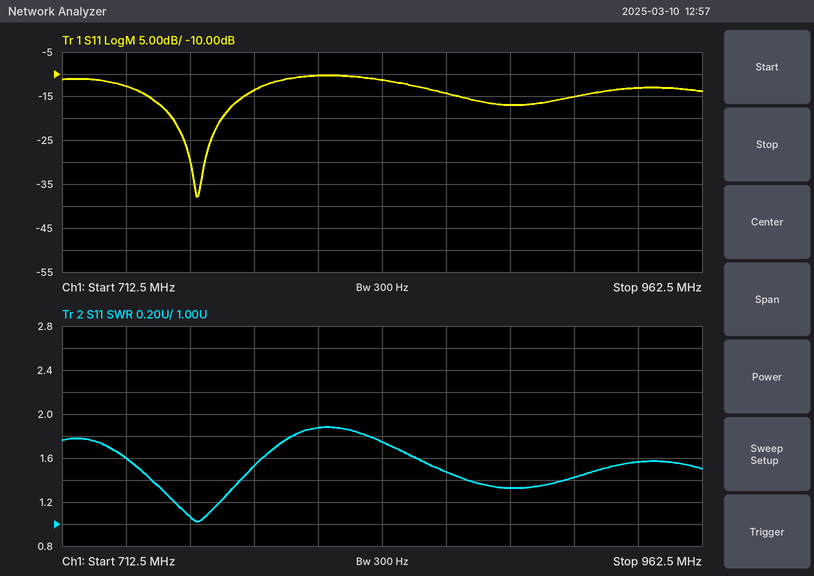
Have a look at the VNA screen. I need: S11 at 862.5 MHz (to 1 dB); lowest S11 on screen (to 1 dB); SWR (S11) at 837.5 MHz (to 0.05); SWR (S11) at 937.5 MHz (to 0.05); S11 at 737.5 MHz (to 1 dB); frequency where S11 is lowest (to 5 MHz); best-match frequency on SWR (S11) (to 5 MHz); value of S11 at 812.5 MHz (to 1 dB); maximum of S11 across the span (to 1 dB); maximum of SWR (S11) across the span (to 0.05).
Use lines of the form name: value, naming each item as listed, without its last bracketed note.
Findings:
S11 at 862.5 MHz: -14 dB
lowest S11 on screen: -38 dB
SWR (S11) at 837.5 MHz: 1.75
SWR (S11) at 937.5 MHz: 1.55
S11 at 737.5 MHz: -13 dB
frequency where S11 is lowest: 765 MHz
best-match frequency on SWR (S11): 765 MHz
value of S11 at 812.5 MHz: -10 dB
maximum of S11 across the span: -10 dB
maximum of SWR (S11) across the span: 1.90
